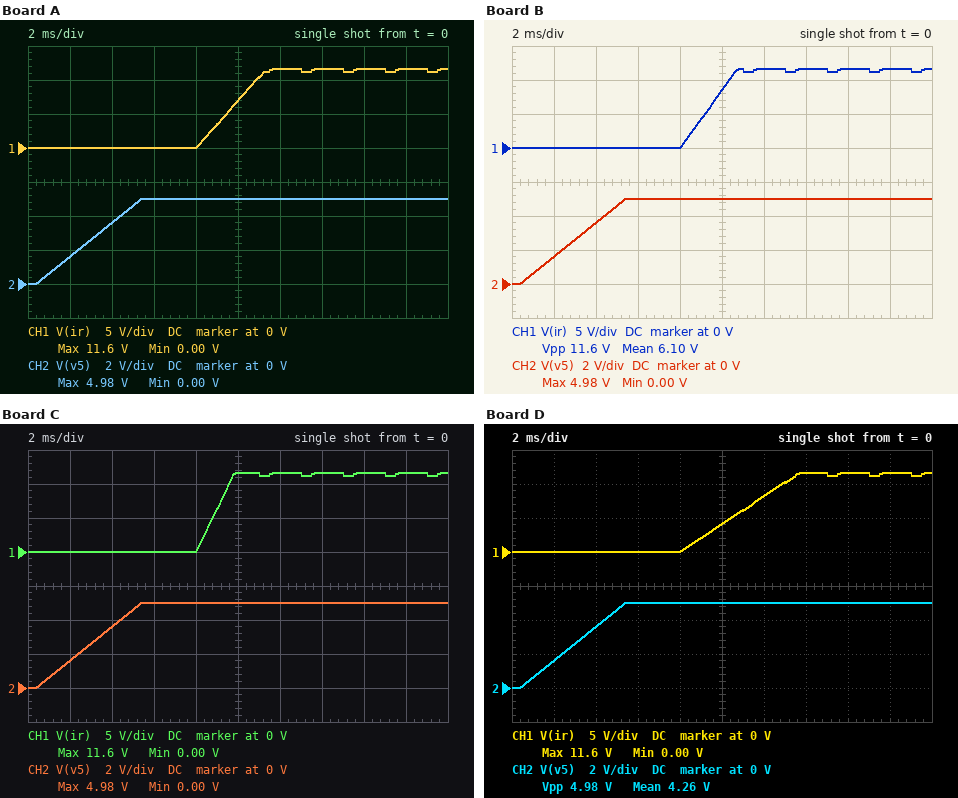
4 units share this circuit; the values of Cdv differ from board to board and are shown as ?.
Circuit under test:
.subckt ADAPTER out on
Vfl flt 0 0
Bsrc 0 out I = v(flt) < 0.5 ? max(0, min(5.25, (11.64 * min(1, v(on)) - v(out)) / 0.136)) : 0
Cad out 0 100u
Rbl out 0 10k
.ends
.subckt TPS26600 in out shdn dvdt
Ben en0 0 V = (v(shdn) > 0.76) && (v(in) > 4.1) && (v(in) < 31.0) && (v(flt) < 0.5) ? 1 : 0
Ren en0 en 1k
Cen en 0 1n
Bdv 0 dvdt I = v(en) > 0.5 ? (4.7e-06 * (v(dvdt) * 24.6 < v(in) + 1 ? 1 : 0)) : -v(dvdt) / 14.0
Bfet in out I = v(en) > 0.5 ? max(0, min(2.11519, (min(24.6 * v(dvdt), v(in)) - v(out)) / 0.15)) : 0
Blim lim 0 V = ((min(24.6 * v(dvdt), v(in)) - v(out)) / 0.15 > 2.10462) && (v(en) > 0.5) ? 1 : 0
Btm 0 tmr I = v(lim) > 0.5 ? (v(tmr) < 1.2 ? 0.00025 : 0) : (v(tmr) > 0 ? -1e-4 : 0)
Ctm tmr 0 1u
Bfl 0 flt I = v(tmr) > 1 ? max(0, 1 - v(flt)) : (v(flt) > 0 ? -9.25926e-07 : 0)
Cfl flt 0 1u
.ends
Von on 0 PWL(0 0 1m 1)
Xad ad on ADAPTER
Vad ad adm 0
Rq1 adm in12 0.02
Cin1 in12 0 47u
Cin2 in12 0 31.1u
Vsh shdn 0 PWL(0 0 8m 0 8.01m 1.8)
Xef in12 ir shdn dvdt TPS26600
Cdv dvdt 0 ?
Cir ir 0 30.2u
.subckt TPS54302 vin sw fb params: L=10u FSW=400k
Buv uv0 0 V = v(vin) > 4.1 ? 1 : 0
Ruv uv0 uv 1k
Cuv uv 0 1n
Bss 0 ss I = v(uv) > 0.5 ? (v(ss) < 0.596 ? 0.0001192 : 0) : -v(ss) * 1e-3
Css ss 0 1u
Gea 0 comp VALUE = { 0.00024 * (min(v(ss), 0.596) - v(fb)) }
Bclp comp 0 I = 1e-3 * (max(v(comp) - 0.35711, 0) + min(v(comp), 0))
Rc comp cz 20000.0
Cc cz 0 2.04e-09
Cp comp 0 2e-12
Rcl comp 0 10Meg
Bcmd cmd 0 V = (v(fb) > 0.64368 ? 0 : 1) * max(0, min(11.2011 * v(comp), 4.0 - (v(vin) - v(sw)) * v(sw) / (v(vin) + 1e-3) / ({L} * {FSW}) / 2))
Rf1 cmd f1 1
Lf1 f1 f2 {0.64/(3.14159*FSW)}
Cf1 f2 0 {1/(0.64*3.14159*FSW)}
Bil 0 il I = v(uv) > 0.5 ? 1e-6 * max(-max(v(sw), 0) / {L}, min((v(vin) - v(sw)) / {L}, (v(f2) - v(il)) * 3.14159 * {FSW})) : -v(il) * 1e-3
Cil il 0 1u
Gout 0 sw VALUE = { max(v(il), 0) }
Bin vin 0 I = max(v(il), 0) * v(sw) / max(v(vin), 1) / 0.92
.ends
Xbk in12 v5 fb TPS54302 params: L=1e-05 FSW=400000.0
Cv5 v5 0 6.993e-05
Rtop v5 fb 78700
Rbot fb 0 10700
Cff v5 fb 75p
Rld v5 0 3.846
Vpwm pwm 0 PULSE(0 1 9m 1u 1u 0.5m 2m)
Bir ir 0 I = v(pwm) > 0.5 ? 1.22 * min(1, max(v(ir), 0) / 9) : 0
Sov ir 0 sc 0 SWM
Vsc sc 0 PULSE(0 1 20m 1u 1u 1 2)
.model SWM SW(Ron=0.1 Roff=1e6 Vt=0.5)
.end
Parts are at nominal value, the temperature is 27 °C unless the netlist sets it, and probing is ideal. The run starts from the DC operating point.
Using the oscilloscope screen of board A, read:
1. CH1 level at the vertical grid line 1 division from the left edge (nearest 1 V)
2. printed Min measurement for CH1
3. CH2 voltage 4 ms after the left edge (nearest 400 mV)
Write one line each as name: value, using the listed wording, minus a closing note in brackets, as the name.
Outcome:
CH1 level at the vertical grid line 1 division from the left edge: 0 V
printed Min measurement for CH1: 0.00 V
CH2 voltage 4 ms after the left edge: 3.6 V
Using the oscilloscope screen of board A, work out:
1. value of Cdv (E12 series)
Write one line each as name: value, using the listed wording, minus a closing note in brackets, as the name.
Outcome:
value of Cdv: 33 nF
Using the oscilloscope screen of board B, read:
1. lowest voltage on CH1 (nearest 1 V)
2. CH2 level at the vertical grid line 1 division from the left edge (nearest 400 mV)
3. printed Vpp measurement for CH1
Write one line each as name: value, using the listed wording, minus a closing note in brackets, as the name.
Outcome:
lowest voltage on CH1: 0 V
CH2 level at the vertical grid line 1 division from the left edge: 1.6 V
printed Vpp measurement for CH1: 11.6 V
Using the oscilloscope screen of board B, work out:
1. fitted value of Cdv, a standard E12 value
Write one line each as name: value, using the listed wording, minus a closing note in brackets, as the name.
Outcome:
fitted value of Cdv, a standard E12 value: 27 nF
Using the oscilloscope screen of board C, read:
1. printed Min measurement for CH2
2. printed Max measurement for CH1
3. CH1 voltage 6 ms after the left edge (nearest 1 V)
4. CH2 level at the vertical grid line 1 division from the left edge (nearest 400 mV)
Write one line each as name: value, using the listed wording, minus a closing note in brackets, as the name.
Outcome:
printed Min measurement for CH2: 0.00 V
printed Max measurement for CH1: 11.6 V
CH1 voltage 6 ms after the left edge: 0 V
CH2 level at the vertical grid line 1 division from the left edge: 1.6 V
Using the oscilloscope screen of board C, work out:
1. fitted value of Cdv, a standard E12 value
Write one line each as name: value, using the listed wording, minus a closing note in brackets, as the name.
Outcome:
fitted value of Cdv, a standard E12 value: 18 nF
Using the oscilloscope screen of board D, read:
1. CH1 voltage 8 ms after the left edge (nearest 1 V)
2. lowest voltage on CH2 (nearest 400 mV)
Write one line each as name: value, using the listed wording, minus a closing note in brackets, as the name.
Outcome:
CH1 voltage 8 ms after the left edge: 0 V
lowest voltage on CH2: 0 V
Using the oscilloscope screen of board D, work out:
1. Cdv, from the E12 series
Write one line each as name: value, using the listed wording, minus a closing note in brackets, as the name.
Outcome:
Cdv, from the E12 series: 56 nF
